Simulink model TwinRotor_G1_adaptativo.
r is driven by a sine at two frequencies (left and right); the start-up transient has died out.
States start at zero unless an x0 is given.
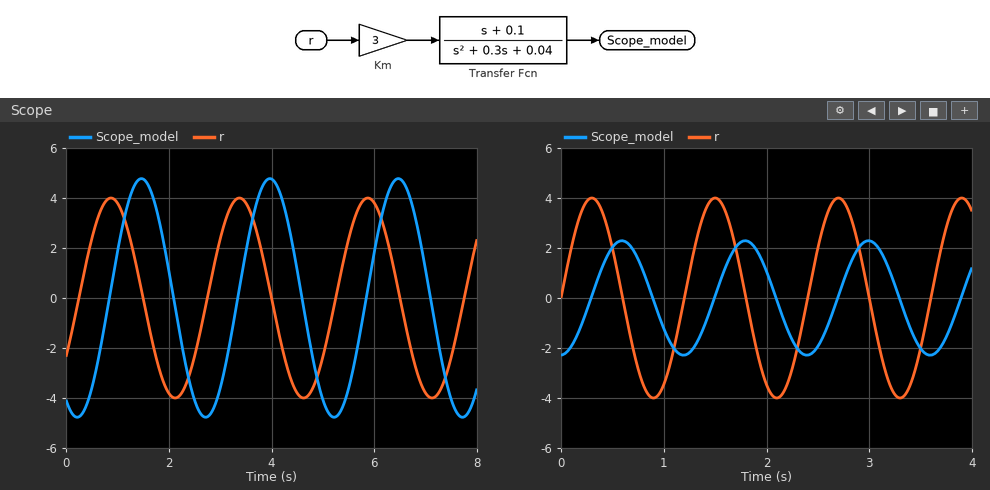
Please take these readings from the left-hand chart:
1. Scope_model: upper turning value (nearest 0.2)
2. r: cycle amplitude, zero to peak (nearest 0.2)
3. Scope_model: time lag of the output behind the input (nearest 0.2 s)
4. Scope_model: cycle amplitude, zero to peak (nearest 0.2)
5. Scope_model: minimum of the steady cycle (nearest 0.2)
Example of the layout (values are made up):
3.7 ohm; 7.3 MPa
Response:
4.8; 4.0; 0.6 s; 4.8; -4.8
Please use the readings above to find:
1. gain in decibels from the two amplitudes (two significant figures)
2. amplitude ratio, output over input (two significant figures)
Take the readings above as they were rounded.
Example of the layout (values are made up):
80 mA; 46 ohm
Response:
1.6 dB; 1.2
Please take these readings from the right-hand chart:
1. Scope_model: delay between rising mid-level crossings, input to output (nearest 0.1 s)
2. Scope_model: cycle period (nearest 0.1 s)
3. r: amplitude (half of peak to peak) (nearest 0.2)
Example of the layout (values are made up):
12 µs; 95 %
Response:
0.3 s; 1.2 s; 4.0
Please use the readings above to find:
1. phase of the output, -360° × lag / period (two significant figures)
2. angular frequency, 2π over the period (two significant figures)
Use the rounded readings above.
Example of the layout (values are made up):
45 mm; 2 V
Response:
-90°; 5.2 rad/s
